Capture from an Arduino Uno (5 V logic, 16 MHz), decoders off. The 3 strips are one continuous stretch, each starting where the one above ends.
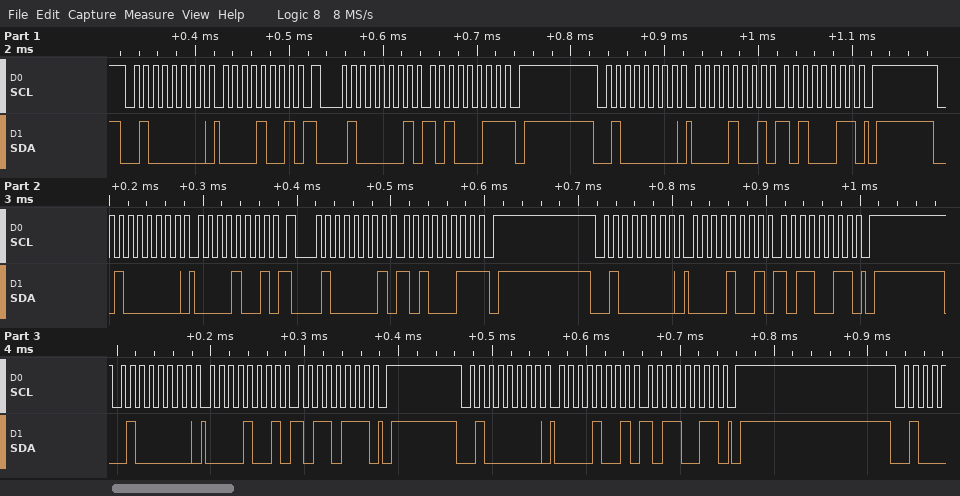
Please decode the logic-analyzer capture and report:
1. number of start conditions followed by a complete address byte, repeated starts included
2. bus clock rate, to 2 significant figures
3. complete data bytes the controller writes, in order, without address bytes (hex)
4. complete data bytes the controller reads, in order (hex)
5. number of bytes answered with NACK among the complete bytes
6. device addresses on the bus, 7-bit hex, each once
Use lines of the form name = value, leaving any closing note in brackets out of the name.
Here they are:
number of start conditions followed by a complete address byte, repeated starts included = 8
bus clock rate, to 2 significant figures = 100 kHz
complete data bytes the controller writes, in order, without address bytes = 09 09 A3 09 09 B3 09 B7 09 B3
complete data bytes the controller reads, in order = A3 A3
number of bytes answered with NACK among the complete bytes = 2
device addresses on the bus, 7-bit hex, each once = 0x20
